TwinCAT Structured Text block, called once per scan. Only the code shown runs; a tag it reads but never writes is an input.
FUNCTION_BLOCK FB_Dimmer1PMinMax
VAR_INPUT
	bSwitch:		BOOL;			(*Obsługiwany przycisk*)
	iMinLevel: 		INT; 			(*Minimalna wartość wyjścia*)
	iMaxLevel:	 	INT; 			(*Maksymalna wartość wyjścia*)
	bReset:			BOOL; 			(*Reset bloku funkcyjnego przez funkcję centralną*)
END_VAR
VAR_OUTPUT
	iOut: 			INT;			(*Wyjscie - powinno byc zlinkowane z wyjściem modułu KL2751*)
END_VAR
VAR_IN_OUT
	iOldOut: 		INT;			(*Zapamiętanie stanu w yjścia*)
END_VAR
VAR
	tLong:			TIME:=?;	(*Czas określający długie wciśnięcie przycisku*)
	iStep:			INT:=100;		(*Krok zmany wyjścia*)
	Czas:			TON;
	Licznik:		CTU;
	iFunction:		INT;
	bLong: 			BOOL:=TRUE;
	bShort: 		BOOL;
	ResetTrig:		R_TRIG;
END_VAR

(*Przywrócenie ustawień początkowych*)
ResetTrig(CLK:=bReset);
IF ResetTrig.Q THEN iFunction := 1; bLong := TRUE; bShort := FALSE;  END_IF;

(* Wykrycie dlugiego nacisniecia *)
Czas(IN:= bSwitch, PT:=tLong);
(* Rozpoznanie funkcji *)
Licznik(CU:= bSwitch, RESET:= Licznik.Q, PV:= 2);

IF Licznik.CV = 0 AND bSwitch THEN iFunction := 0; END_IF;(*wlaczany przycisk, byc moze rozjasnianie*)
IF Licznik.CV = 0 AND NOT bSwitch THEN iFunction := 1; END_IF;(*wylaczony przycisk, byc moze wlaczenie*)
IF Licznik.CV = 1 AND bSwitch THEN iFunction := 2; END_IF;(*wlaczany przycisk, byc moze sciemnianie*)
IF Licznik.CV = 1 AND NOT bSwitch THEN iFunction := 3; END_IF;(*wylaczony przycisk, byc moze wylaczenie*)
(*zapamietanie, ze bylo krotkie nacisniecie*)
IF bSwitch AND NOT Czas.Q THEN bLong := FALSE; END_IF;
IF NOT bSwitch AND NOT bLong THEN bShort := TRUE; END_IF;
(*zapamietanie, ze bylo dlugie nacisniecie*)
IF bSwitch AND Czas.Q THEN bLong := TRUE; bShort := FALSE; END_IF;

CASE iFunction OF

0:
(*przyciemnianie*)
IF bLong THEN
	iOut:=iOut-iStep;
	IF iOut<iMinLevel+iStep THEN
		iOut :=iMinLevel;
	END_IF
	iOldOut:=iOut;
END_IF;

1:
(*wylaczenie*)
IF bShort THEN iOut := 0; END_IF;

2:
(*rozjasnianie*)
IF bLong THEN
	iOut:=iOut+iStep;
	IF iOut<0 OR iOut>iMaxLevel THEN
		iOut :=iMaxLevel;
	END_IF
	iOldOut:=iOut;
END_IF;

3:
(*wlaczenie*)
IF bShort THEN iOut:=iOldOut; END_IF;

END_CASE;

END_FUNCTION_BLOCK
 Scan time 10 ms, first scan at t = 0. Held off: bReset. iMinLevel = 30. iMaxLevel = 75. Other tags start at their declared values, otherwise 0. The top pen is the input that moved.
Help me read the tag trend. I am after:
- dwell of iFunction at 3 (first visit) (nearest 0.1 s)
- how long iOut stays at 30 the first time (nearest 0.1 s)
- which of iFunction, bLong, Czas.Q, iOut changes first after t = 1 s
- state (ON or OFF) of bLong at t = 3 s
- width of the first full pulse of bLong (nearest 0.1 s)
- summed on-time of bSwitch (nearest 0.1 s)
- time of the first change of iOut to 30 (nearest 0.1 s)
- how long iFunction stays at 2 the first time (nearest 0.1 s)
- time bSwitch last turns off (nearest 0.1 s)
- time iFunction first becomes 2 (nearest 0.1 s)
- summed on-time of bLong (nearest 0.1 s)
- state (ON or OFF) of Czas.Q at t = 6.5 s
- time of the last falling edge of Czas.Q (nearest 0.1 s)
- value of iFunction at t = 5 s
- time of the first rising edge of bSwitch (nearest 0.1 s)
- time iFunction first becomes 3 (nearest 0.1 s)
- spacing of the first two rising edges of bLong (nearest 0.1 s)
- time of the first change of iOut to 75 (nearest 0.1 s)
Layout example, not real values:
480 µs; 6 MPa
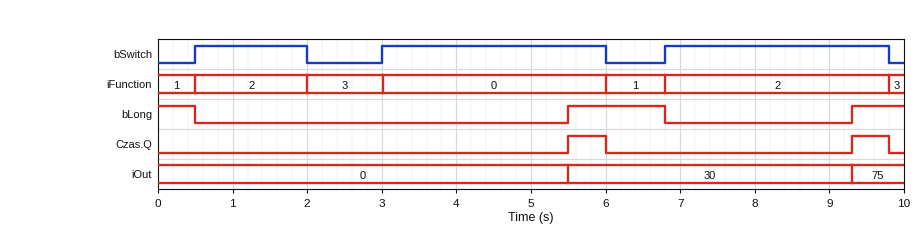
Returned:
1.0 s; 3.8 s; iFunction; OFF; 1.3 s; 7.5 s; 5.5 s; 1.5 s; 9.8 s; 0.5 s; 2.5 s; OFF; 9.8 s; 0; 0.5 s; 2.0 s; 3.8 s; 9.3 s
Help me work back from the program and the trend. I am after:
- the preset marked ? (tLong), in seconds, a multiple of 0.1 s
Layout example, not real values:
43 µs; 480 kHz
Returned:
2.5 s
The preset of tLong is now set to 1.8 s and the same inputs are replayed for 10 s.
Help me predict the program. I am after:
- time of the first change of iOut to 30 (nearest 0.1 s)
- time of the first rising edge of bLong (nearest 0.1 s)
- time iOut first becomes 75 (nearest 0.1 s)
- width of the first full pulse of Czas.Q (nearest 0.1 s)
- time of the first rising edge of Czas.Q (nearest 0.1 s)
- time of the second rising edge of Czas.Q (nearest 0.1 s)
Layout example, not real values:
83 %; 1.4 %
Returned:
4.8 s; 4.8 s; 8.6 s; 1.2 s; 4.8 s; 8.6 s
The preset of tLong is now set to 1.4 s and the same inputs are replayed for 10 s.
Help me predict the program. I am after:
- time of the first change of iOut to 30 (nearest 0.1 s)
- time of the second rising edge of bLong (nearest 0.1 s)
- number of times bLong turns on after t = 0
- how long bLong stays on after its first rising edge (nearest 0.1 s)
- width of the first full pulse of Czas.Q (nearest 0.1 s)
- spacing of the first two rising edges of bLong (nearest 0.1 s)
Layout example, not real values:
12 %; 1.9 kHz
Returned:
4.4 s; 4.4 s; 3; 1.1 s; 0.1 s; 2.5 s
